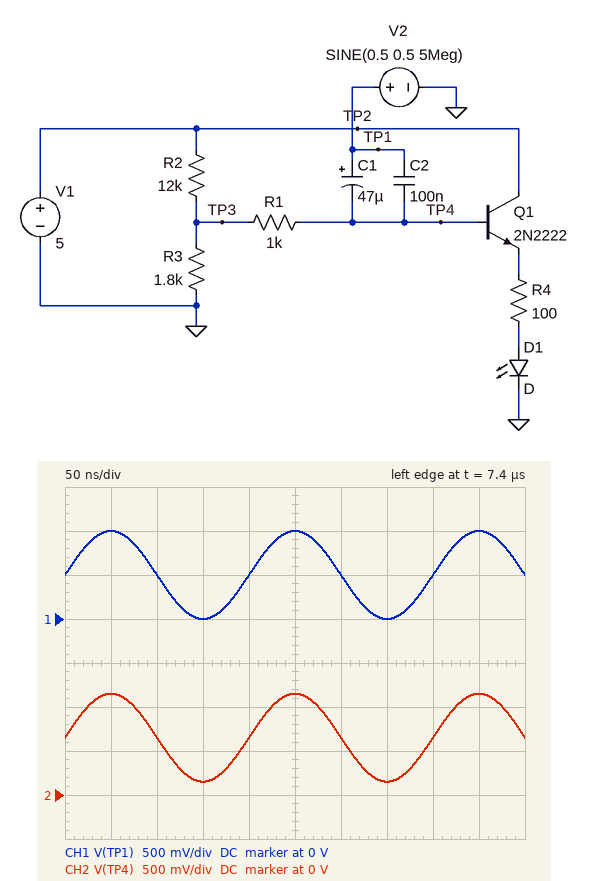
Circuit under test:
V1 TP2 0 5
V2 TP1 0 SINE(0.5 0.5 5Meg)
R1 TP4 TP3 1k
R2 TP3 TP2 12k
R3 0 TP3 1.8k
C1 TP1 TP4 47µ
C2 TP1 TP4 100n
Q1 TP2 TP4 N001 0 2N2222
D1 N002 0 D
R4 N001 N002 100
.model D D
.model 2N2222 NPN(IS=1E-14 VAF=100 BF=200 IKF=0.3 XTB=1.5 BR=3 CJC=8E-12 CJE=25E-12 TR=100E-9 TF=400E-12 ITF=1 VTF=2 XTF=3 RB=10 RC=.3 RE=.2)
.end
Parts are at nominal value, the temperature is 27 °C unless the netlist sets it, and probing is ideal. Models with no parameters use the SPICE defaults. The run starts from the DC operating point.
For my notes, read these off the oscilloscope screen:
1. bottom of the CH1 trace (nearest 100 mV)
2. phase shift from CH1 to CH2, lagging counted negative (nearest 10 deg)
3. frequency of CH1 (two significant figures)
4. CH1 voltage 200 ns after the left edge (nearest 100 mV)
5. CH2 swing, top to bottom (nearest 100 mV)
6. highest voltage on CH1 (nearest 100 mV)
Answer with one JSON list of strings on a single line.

["0 V", "0 deg", "5.0 MHz", "500 mV", "1.0 V", "1.0 V"]
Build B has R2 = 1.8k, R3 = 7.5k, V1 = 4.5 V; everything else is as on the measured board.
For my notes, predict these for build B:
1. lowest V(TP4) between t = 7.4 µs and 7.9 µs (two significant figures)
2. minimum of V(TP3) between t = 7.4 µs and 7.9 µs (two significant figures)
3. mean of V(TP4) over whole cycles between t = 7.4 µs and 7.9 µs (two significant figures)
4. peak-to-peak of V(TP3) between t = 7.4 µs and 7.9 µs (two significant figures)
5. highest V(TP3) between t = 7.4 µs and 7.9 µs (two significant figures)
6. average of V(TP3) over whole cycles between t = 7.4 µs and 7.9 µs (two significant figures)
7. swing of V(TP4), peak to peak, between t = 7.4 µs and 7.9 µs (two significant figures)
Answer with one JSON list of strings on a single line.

["2.9 V", "3.2 V", "3.4 V", "590 mV", "3.8 V", "3.5 V", "1.0 V"]
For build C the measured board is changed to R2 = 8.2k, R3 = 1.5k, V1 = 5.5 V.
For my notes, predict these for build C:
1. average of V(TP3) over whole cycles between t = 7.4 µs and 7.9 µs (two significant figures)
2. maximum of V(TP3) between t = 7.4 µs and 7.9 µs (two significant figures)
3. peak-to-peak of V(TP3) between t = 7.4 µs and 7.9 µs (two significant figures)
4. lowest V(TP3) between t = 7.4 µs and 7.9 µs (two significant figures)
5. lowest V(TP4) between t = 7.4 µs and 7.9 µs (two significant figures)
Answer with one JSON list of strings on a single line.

["850 mV", "1.1 V", "560 mV", "570 mV", "350 mV"]
